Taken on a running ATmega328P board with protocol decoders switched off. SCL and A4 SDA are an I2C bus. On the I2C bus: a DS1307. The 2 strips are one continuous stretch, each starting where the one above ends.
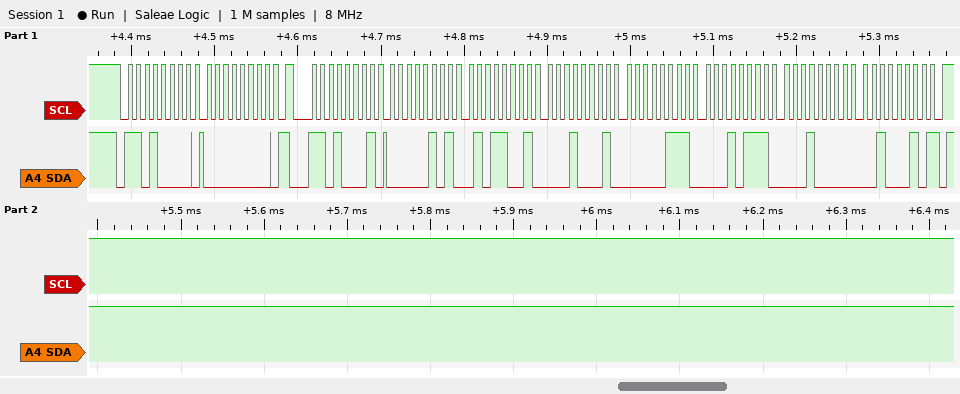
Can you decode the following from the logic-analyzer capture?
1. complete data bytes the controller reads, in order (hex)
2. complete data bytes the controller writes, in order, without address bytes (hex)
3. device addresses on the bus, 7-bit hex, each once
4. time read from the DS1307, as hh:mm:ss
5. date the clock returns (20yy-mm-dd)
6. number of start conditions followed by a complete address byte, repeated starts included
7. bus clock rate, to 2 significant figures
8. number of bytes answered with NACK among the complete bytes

05 59 11 07 17 10 22
00
0x68
11:59:05
2022-10-17
2
100 kHz
1
